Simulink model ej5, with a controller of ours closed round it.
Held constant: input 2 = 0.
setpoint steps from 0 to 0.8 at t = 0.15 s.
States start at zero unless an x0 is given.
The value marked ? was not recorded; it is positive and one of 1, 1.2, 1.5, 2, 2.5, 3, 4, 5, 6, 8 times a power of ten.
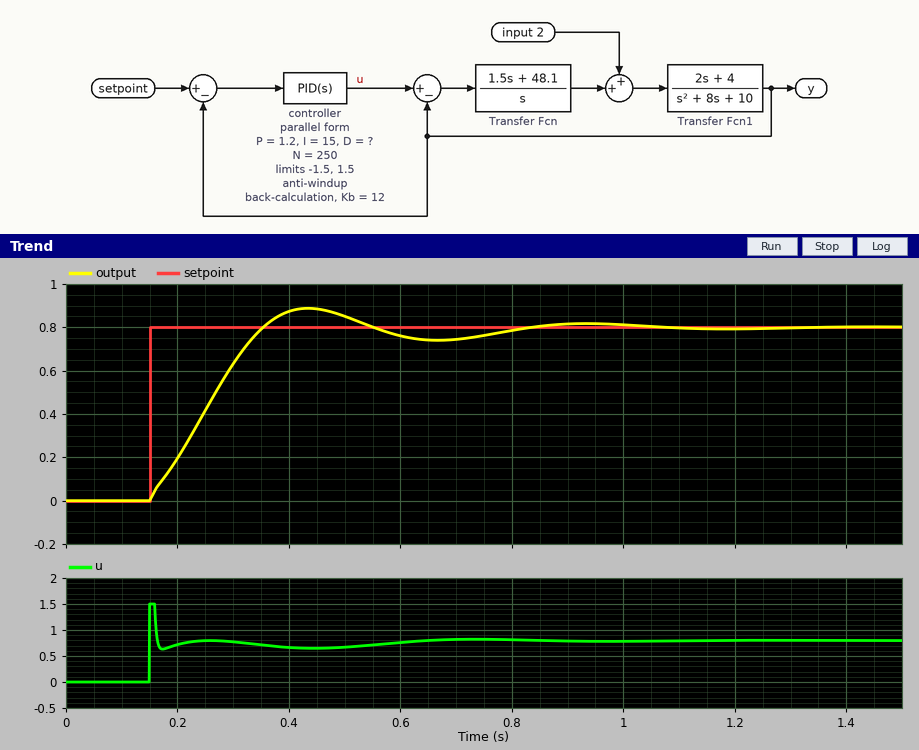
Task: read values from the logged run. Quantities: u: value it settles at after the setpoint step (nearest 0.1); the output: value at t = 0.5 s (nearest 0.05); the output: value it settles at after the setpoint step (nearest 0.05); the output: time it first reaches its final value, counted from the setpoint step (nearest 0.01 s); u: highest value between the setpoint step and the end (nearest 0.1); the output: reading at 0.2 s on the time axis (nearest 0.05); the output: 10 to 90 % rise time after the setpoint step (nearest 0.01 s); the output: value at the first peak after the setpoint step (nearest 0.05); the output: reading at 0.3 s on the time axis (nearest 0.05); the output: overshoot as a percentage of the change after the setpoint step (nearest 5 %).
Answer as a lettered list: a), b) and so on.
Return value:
a) 0.8
b) 0.85
c) 0.80
d) 0.20 s
e) 1.5
f) 0.20
g) 0.16 s
h) 0.90
i) 0.65
j) 10 %
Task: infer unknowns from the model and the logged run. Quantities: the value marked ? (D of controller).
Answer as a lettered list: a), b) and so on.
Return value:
a) 0.05
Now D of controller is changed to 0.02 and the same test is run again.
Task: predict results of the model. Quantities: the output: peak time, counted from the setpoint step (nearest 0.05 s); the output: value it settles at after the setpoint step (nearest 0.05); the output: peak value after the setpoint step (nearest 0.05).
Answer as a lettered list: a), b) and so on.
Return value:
a) 0.25 s
b) 0.80
c) 0.95
